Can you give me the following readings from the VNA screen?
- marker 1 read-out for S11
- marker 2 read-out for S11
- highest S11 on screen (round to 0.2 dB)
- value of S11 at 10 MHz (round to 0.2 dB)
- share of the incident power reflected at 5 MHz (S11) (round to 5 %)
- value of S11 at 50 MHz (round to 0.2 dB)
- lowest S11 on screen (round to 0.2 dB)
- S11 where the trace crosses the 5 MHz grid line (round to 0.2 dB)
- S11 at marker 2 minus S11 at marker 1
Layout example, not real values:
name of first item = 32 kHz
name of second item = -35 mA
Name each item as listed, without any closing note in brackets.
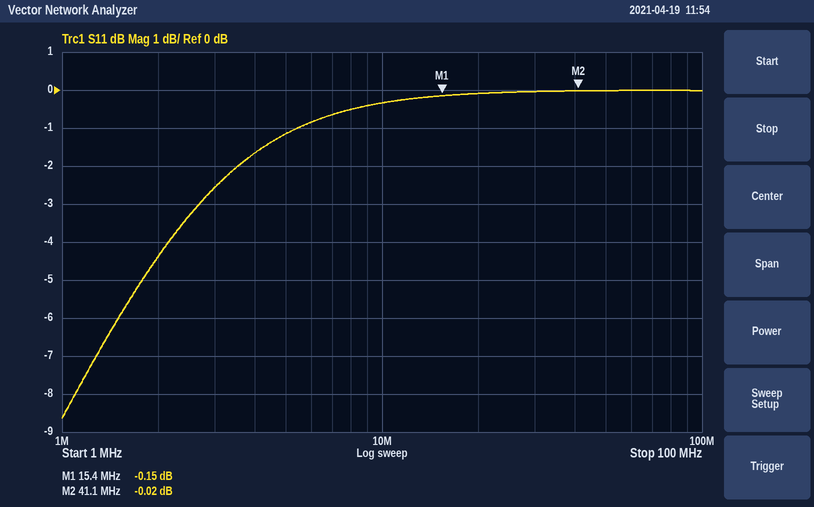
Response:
marker 1 read-out for S11 = -0.15 dB
marker 2 read-out for S11 = -0.02 dB
highest S11 on screen = 0.0 dB
value of S11 at 10 MHz = -0.4 dB
share of the incident power reflected at 5 MHz (S11) = 75 %
value of S11 at 50 MHz = 0.0 dB
lowest S11 on screen = -8.6 dB
S11 where the trace crosses the 5 MHz grid line = -1.2 dB
S11 at marker 2 minus S11 at marker 1 = 0.13 dB
